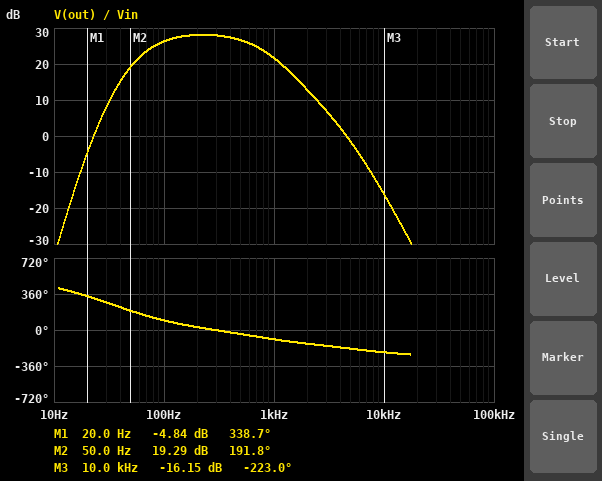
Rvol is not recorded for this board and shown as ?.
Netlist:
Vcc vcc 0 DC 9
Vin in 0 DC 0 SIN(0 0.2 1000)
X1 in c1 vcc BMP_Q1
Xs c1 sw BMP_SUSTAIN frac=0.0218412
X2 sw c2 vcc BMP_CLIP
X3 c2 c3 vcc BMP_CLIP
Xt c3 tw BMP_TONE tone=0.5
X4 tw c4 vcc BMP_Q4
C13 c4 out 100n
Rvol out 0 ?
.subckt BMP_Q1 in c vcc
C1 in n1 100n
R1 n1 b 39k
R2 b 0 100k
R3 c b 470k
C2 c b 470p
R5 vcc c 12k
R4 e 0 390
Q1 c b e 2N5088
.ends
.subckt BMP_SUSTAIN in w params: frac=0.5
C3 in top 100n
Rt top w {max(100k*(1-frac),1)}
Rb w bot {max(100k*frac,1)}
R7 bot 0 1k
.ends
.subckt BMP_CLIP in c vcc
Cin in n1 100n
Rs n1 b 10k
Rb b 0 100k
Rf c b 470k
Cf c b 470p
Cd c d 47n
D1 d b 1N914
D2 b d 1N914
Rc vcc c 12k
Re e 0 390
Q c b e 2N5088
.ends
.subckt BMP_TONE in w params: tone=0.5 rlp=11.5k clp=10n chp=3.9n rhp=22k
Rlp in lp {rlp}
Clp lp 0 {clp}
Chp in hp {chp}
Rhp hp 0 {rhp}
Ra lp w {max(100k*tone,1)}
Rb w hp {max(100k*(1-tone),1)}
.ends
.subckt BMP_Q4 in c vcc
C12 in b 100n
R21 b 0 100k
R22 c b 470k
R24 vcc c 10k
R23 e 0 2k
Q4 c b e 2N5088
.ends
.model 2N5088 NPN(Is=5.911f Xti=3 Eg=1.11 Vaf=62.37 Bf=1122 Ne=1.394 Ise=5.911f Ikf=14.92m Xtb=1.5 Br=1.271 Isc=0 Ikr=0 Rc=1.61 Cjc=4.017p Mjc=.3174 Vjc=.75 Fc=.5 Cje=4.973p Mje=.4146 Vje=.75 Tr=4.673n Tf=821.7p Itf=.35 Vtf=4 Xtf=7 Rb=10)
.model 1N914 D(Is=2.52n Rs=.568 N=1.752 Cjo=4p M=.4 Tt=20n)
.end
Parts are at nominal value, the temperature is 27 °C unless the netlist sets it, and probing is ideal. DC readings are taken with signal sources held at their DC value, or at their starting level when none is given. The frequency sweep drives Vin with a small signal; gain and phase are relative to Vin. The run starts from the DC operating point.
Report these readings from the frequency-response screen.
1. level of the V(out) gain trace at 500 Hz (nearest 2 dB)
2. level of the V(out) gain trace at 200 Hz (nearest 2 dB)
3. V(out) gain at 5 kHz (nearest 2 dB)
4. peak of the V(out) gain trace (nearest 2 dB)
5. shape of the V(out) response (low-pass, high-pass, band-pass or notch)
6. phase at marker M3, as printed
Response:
26 dB
28 dB
-2 dB
28 dB
band-pass
-223.0 deg
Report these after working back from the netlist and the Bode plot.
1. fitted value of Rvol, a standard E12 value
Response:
33 kΩ
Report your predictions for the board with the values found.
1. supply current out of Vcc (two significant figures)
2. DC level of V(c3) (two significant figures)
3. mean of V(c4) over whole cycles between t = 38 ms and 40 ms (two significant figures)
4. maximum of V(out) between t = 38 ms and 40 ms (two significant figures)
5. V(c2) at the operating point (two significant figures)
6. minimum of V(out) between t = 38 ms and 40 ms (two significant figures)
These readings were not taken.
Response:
1.3 mA
4.6 V
6.5 V
400 mV
4.7 V
-400 mV
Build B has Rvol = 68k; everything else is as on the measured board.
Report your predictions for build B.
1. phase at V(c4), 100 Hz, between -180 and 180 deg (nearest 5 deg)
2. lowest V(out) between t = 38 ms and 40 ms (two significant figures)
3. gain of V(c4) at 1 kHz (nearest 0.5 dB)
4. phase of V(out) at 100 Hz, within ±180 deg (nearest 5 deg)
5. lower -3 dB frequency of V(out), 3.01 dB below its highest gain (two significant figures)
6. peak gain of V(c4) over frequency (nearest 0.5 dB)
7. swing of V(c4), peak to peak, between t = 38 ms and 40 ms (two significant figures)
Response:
75 deg
-450 mV
22.5 dB
85 deg
77 Hz
29.0 dB
910 mV
